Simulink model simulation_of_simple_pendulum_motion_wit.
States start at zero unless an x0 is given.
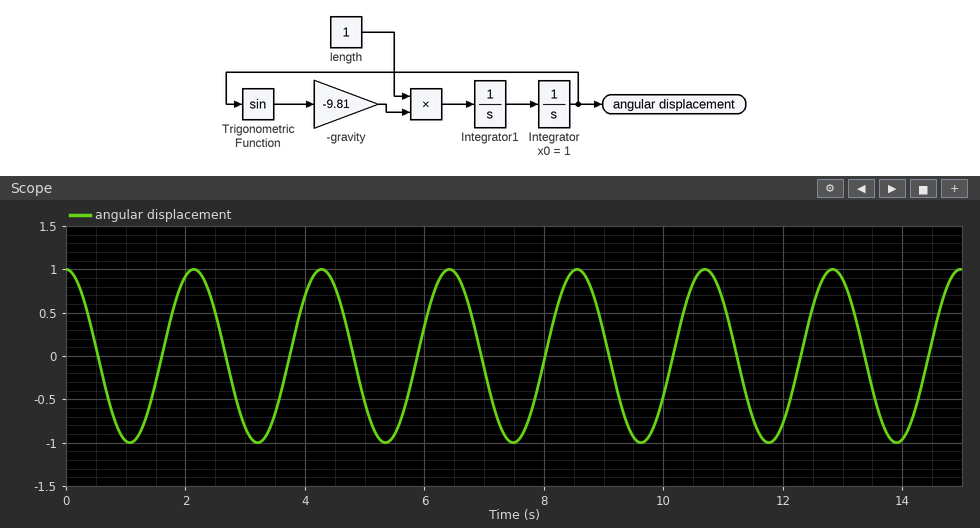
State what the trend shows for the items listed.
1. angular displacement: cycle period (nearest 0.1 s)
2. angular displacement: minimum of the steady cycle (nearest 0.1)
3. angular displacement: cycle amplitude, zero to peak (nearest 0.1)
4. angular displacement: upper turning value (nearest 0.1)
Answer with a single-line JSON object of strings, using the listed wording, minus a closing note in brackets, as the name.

{"angular displacement: cycle period": "2.1 s", "angular displacement: minimum of the steady cycle": "-1.0", "angular displacement: cycle amplitude, zero to peak": "1.0", "angular displacement: upper turning value": "1.0"}
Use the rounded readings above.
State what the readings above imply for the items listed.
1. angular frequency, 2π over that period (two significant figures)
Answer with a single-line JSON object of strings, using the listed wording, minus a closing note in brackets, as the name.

{"angular frequency, 2π over that period": "3.0 rad/s"}
